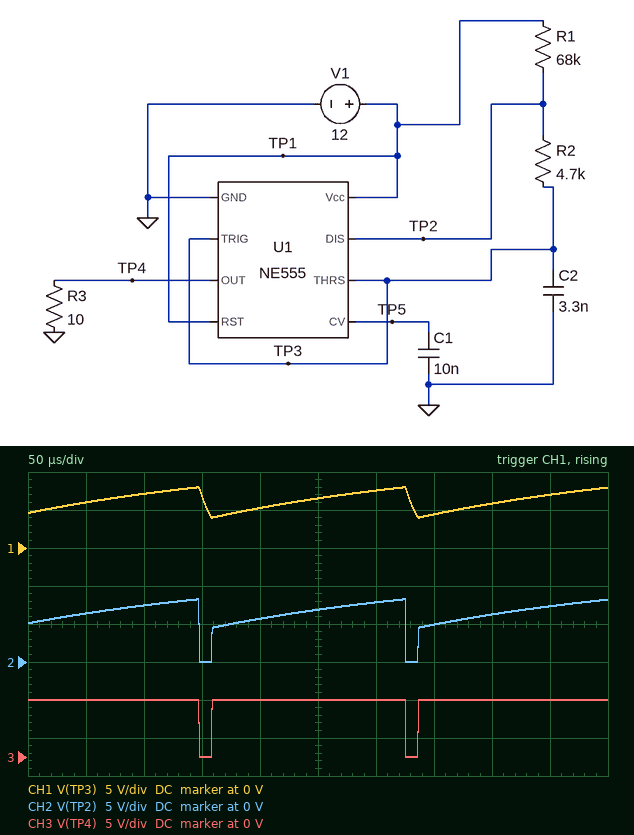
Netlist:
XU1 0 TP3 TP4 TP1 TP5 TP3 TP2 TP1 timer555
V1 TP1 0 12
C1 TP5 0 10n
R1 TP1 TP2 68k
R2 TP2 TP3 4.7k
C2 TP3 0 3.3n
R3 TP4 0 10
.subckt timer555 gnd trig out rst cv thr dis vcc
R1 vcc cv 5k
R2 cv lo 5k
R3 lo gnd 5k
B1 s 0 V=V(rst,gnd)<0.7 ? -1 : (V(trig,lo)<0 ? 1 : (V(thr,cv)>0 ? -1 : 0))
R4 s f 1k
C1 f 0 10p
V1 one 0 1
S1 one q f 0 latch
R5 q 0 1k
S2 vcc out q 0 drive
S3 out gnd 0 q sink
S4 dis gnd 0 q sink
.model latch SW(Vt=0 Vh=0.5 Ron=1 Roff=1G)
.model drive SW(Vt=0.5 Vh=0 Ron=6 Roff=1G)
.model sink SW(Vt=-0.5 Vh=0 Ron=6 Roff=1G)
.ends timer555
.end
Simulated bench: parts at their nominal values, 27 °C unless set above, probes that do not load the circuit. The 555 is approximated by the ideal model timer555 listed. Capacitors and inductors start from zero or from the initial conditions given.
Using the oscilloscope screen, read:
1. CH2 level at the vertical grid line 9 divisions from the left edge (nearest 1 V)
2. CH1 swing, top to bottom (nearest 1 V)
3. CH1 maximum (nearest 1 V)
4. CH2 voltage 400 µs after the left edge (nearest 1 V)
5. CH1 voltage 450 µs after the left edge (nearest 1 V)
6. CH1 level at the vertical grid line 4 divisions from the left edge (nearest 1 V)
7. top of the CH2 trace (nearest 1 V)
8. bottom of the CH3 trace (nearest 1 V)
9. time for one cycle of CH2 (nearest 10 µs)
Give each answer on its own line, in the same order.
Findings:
7 V
4 V
8 V
6 V
7 V
5 V
8 V
0 V
180 µs
